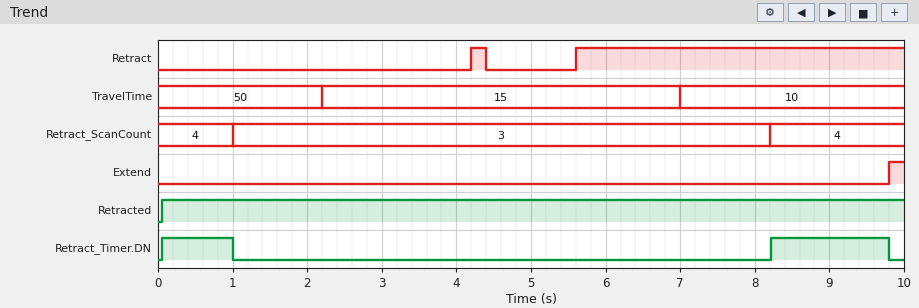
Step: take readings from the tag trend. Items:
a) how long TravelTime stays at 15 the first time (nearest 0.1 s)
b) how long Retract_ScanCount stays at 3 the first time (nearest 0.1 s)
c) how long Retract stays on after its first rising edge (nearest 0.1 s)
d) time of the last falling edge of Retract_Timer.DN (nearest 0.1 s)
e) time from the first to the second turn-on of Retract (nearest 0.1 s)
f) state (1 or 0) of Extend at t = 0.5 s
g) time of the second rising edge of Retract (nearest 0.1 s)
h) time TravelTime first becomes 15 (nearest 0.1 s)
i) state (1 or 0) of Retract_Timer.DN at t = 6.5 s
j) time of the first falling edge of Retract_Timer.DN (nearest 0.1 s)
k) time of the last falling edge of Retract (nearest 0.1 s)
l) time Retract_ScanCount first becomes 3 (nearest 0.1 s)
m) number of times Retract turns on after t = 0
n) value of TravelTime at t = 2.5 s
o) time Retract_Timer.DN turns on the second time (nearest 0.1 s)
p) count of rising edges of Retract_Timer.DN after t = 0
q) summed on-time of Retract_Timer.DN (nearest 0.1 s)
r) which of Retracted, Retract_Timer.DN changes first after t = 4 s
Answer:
4.8 s
7.2 s
0.2 s
9.8 s
1.4 s
0
5.6 s
2.2 s
0
1.0 s
4.4 s
1.0 s
2
15
8.2 s
2
2.5 s
Retract_Timer.DN
